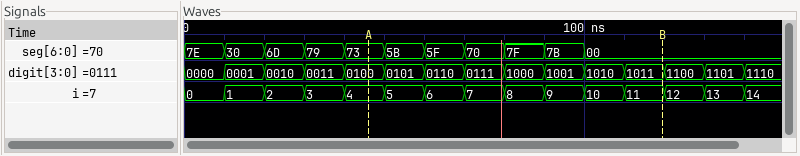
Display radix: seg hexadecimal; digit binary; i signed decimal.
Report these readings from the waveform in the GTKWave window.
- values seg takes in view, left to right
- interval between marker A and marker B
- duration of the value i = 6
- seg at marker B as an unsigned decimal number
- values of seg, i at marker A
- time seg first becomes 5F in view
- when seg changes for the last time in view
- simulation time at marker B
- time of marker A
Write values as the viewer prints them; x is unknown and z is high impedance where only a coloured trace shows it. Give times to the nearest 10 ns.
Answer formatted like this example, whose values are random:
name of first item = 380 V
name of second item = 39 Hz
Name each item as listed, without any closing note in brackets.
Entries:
values seg takes in view, left to right = 7E, 30, 6D, 79, 73, 5B, 5F, 70, 7F, 7B, 00
interval between marker A and marker B = 70 ns
duration of the value i = 6 = 10 ns
seg at marker B as an unsigned decimal number = 0
values of seg, i at marker A = seg=73, i=4
time seg first becomes 5F in view = 60 ns
when seg changes for the last time in view = 100 ns
simulation time at marker B = 120 ns
time of marker A = 50 ns
